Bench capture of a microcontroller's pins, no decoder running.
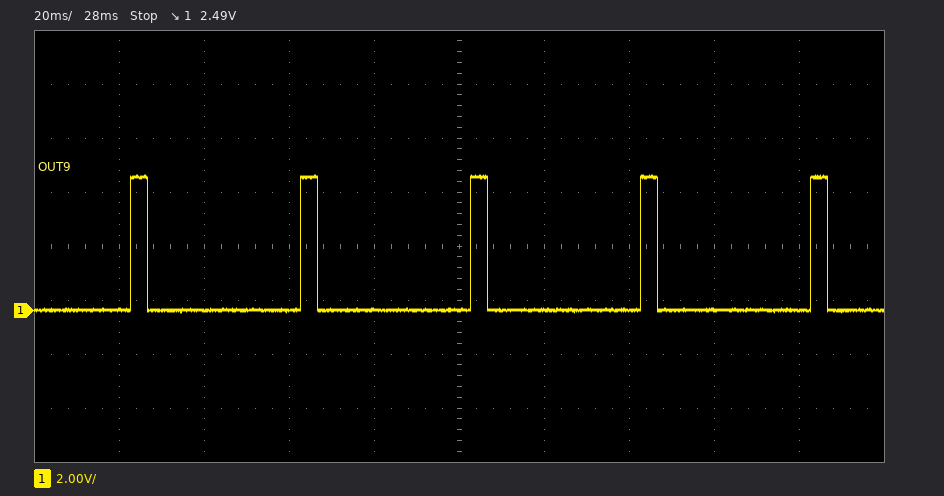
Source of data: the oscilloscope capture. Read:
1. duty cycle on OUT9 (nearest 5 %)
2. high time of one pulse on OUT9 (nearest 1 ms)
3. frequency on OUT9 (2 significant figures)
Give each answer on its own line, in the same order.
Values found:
10 %
4 ms
25 Hz
